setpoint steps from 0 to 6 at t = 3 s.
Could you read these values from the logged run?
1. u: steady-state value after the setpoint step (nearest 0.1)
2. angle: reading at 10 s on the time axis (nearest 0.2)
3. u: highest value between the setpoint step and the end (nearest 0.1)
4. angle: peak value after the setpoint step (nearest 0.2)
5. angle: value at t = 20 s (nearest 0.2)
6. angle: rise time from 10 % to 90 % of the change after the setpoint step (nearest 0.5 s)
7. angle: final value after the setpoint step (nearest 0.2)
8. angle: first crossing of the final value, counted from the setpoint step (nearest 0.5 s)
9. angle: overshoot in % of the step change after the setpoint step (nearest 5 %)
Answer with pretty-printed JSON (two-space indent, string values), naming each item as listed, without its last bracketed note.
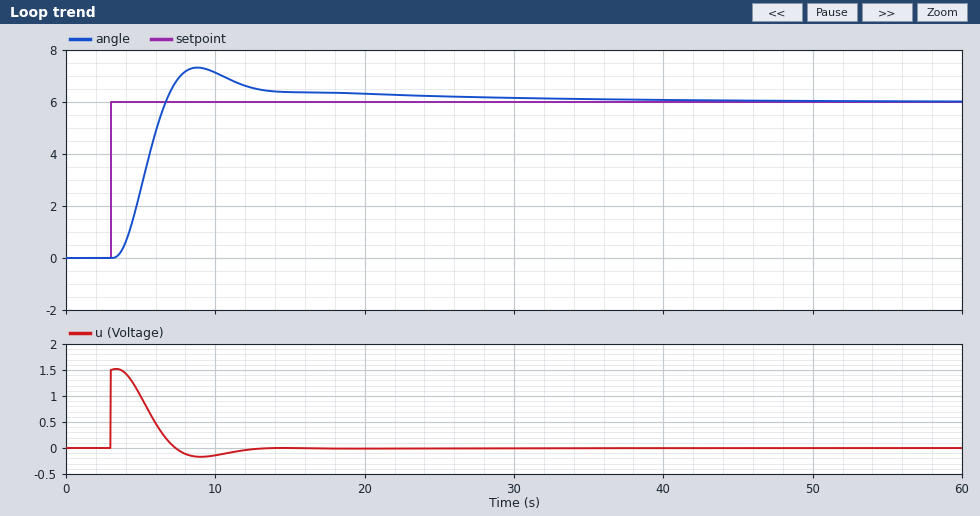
{
  "u: steady-state value after the setpoint step": "0.0",
  "angle: reading at 10 s on the time axis": "7.2",
  "u: highest value between the setpoint step and the end": "1.5",
  "angle: peak value after the setpoint step": "7.4",
  "angle: value at t = 20 s": "6.4",
  "angle: rise time from 10 % to 90 % of the change after the setpoint step": "2.5 s",
  "angle: final value after the setpoint step": "6.0",
  "angle: first crossing of the final value, counted from the setpoint step": "3.5 s",
  "angle: overshoot in % of the step change after the setpoint step": "20 %"
}
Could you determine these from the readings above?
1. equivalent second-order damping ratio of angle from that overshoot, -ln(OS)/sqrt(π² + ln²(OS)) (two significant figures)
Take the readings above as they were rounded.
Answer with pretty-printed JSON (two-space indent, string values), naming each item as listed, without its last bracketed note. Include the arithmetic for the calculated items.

{
  "equivalent second-order damping ratio of angle from that overshoot, -ln(OS)/sqrt(π² + ln²(OS))": "ln(0.2) = -1.609; 1.609 / sqrt(9.870 + 2.590) = 0.46"
}
